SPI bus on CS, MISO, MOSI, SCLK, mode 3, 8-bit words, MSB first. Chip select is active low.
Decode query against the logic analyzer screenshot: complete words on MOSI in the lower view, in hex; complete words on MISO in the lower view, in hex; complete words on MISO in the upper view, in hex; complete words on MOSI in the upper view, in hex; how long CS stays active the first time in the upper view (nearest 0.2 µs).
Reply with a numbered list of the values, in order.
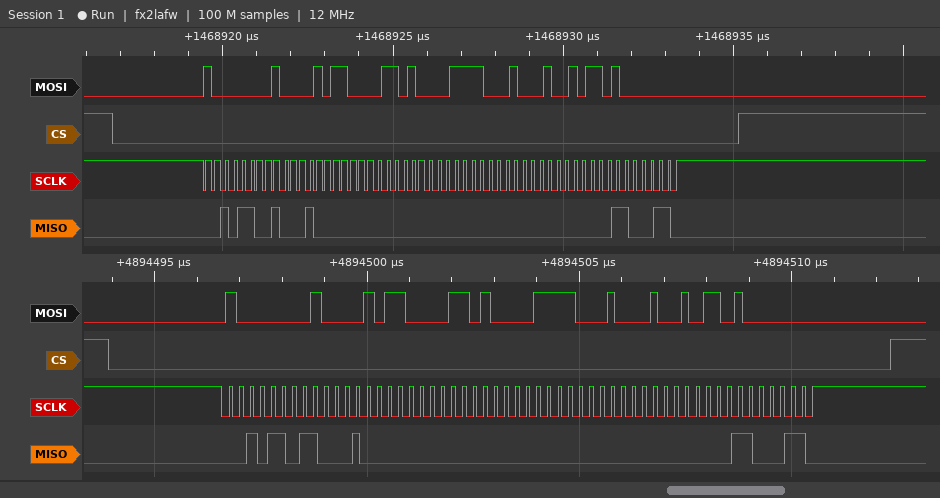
1. 80, 85, 86, 87, 88, 96, 80
2. 2D, 88, 00, 00, 00, 00, C6
3. 2C, 88, 00, 00, 00, 00, C6
4. 80, 85, 86, 87, 88, 96, 80
5. 18.4 µs
